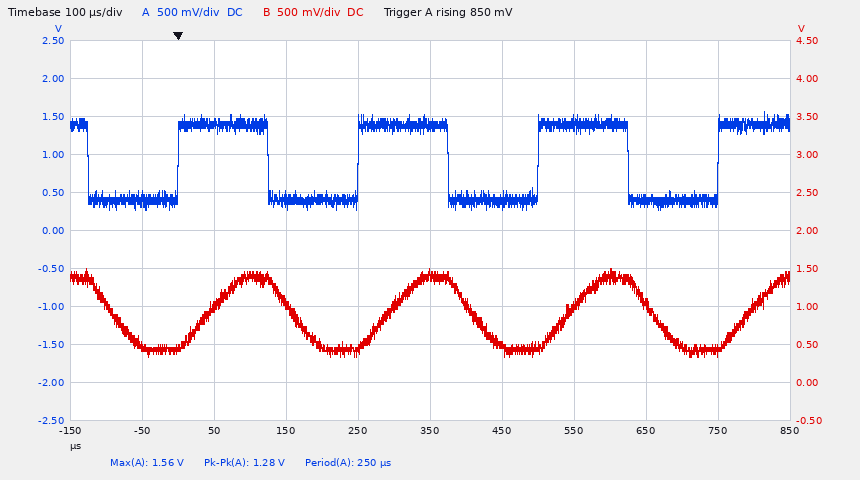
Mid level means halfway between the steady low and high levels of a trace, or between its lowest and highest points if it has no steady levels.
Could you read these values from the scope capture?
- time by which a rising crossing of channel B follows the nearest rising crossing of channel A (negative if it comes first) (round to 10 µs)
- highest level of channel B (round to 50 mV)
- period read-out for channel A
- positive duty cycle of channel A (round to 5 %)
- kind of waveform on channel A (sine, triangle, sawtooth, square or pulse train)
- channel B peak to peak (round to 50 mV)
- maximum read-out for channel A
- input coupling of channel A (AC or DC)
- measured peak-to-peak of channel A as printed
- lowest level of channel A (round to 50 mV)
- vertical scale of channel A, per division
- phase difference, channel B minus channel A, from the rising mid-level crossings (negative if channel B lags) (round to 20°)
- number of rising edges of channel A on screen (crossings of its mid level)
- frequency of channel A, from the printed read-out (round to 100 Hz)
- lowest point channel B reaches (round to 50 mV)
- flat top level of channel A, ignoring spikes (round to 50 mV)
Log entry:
+40 µs
1.50 V
250 µs
50 %
square
1.15 V
1.56 V
DC
1.28 V
300 mV
500 mV
-60°
4
4.0 kHz
350 mV
1.40 V
